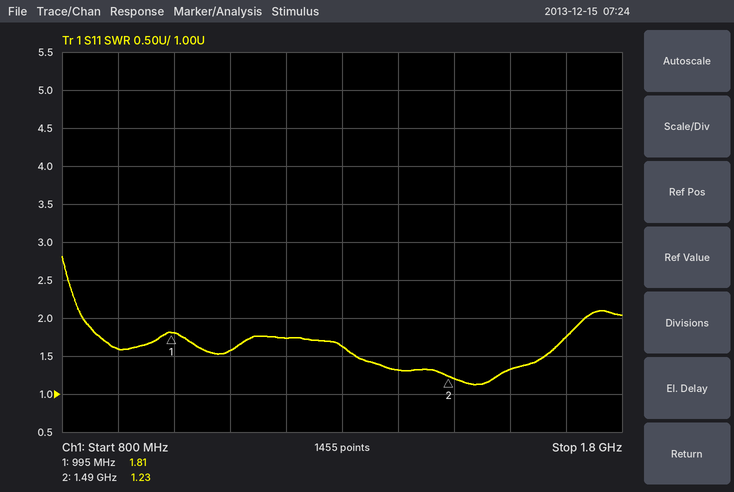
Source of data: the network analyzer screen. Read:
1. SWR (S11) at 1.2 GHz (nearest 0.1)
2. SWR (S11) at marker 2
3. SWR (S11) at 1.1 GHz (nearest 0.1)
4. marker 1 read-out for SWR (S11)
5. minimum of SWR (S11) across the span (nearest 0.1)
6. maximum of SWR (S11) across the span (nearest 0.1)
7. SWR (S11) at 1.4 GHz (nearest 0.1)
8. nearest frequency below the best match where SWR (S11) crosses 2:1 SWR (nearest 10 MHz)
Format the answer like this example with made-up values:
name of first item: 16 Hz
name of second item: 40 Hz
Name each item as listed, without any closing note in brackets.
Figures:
SWR (S11) at 1.2 GHz: 1.7
SWR (S11) at marker 2: 1.23
SWR (S11) at 1.1 GHz: 1.6
marker 1 read-out for SWR: 1.81
minimum of SWR (S11) across the span: 1.1
maximum of SWR (S11) across the span: 2.8
SWR (S11) at 1.4 GHz: 1.3
nearest frequency below the best match where SWR (S11) crosses 2:1 SWR: 840 MHz
